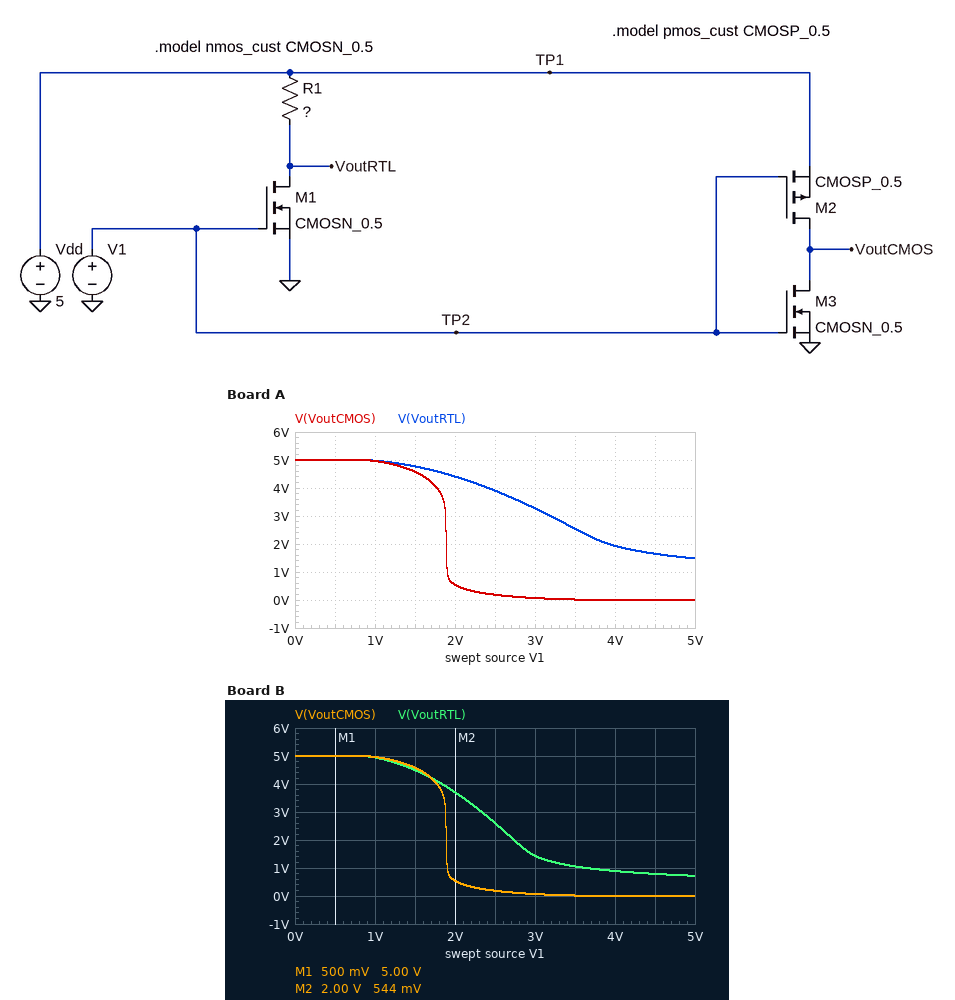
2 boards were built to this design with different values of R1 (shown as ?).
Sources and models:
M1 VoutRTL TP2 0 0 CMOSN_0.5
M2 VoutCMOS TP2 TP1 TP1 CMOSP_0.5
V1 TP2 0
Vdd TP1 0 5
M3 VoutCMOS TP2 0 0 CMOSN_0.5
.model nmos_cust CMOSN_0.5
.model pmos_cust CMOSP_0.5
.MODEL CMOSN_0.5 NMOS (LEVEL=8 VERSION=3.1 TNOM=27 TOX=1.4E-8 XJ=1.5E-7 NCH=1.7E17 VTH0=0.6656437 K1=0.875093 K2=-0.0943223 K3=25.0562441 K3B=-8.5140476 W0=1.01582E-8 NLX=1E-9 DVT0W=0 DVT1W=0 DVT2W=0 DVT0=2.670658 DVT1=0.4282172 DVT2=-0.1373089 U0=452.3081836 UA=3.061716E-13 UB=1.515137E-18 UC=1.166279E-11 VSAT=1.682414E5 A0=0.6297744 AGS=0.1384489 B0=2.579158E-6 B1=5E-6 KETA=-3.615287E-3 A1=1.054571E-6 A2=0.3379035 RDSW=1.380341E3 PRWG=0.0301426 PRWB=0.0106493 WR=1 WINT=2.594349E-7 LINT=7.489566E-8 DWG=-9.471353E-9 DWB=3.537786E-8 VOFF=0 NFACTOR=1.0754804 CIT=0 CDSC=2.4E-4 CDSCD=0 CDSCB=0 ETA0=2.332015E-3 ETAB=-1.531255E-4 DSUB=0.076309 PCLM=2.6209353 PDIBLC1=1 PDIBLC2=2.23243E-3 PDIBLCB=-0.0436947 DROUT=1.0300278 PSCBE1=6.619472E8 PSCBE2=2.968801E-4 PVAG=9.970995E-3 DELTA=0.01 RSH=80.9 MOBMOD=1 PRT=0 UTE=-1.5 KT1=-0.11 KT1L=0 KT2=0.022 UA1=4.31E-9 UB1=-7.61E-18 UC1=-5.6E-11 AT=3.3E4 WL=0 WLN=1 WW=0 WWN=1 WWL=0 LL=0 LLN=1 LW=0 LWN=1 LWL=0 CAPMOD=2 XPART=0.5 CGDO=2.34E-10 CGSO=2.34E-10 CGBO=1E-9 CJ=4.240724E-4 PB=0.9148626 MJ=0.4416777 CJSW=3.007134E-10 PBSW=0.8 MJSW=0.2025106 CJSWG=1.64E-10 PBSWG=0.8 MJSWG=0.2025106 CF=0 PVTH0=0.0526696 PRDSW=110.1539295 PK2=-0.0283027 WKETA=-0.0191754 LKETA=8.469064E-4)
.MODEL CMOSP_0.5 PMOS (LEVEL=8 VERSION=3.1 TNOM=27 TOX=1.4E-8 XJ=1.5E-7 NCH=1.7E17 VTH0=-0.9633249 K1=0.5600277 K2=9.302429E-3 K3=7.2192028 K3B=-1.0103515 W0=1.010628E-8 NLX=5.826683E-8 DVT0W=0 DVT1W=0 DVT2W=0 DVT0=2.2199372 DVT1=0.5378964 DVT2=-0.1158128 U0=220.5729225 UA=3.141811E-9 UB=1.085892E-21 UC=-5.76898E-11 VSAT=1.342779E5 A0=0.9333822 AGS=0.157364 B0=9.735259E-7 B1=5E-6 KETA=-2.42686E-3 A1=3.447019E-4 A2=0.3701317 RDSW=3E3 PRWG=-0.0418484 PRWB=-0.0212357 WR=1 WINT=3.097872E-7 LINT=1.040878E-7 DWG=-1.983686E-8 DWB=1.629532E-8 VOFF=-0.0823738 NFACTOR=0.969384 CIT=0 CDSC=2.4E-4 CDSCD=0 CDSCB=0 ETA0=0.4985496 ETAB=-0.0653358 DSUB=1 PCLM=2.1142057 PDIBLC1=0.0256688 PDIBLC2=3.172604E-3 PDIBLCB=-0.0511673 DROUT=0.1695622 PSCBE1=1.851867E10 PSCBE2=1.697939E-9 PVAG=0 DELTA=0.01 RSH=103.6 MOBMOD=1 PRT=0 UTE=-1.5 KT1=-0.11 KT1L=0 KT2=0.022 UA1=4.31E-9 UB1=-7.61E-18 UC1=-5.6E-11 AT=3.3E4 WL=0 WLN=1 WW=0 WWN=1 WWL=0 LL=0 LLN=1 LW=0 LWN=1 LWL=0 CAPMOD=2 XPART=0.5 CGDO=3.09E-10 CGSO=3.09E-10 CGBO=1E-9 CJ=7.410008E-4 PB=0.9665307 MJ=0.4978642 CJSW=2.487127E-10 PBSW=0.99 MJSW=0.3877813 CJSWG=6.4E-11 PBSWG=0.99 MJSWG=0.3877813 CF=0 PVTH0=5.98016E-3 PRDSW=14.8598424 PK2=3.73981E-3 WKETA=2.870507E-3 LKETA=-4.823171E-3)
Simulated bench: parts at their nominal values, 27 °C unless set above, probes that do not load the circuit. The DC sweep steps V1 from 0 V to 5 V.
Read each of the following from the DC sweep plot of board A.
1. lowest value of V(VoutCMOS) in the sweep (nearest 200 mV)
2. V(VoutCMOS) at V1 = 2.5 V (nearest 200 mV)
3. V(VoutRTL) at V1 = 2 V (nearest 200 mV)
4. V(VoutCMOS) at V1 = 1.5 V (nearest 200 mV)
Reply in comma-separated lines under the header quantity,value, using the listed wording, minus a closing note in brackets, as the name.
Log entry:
quantity,value
lowest value of V(VoutCMOS) in the sweep,0 V
V(VoutCMOS) at V1 = 2.5 V,200 mV
V(VoutRTL) at V1 = 2 V,4.4 V
V(VoutCMOS) at V1 = 1.5 V,4.6 V
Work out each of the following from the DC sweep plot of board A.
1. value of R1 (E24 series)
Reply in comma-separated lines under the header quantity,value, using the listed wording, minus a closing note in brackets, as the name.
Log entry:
quantity,value
value of R1,10 kΩ
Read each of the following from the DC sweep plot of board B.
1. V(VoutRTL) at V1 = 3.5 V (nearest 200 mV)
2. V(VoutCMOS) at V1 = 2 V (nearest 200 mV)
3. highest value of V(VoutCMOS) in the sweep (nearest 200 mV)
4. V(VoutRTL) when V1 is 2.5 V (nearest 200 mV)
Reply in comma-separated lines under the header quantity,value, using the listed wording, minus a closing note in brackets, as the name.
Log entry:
quantity,value
V(VoutRTL) at V1 = 3.5 V,1.0 V
V(VoutCMOS) at V1 = 2 V,600 mV
highest value of V(VoutCMOS) in the sweep,5.0 V
V(VoutRTL) when V1 is 2.5 V,2.6 V
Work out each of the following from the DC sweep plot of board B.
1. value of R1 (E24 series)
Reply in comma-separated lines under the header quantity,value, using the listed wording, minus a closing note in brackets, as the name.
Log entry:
quantity,value
value of R1,22 kΩ
